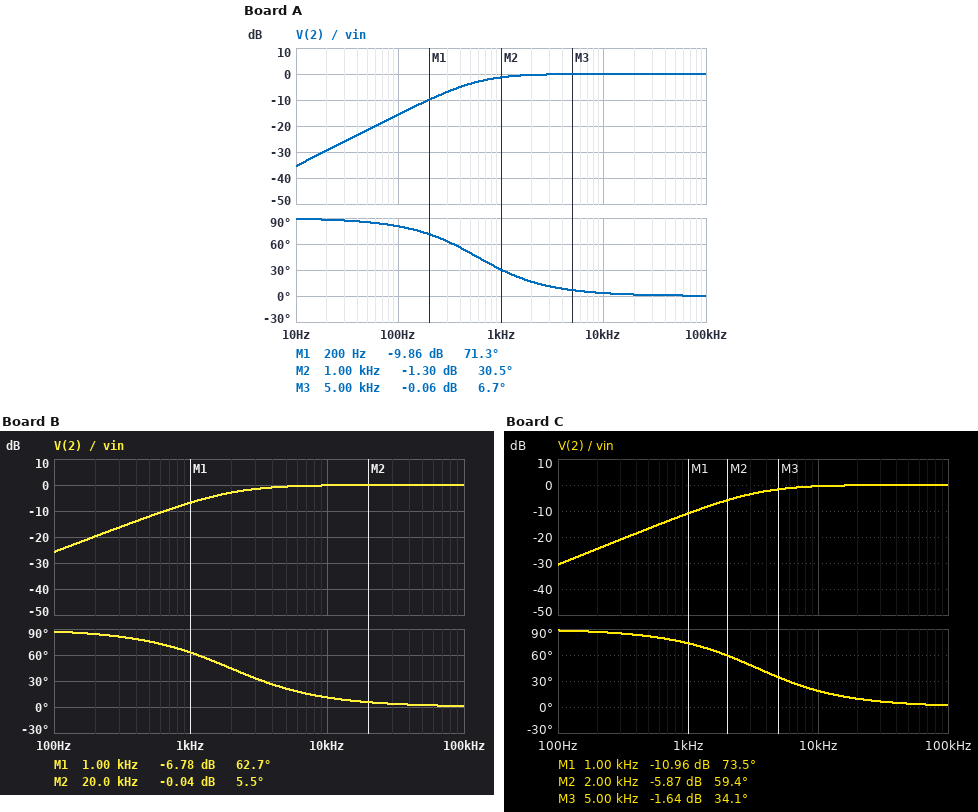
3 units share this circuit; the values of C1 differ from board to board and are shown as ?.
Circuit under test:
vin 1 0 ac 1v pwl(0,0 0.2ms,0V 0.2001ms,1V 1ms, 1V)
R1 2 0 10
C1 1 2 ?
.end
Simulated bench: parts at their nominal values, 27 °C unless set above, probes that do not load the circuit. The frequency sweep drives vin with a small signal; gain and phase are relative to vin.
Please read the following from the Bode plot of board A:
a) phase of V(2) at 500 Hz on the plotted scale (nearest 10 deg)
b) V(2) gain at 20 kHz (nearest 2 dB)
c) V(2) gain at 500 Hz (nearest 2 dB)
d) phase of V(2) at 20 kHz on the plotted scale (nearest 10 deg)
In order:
50 deg
0 dB
-4 dB
0 deg
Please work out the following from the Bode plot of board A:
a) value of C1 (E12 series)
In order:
27 µF
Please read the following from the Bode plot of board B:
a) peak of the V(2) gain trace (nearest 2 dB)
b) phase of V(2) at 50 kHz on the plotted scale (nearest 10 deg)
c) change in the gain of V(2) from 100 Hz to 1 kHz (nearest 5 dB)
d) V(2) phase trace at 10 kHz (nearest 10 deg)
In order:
0 dB
0 deg
20 dB
10 deg
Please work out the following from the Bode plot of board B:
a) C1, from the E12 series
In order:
8.2 µF
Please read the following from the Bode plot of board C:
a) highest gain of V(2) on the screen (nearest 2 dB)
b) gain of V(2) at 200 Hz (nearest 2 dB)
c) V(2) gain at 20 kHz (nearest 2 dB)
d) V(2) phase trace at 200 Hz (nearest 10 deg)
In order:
0 dB
-24 dB
0 dB
90 deg
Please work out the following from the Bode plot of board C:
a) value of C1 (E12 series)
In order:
4.7 µF
